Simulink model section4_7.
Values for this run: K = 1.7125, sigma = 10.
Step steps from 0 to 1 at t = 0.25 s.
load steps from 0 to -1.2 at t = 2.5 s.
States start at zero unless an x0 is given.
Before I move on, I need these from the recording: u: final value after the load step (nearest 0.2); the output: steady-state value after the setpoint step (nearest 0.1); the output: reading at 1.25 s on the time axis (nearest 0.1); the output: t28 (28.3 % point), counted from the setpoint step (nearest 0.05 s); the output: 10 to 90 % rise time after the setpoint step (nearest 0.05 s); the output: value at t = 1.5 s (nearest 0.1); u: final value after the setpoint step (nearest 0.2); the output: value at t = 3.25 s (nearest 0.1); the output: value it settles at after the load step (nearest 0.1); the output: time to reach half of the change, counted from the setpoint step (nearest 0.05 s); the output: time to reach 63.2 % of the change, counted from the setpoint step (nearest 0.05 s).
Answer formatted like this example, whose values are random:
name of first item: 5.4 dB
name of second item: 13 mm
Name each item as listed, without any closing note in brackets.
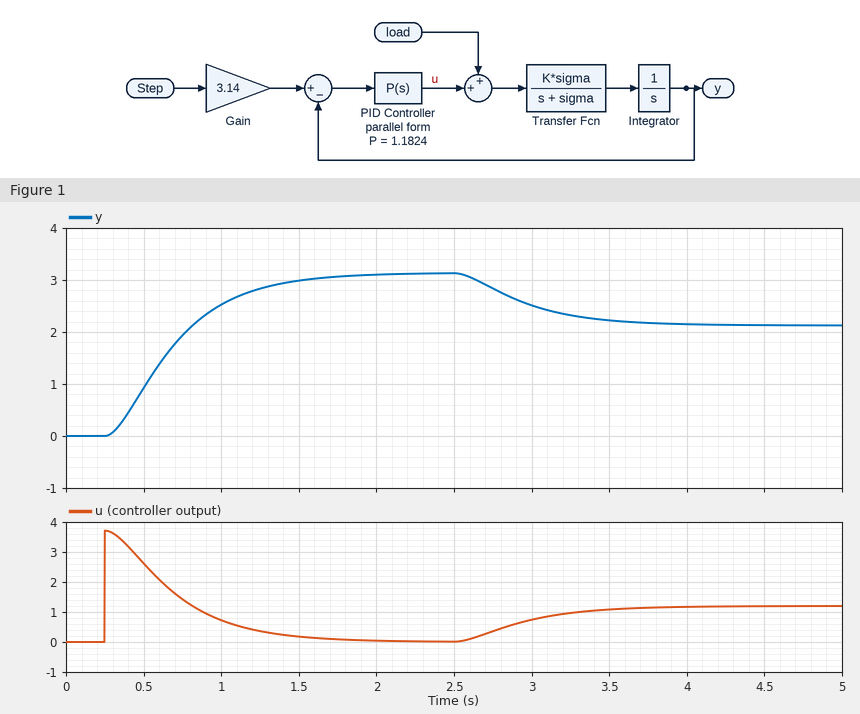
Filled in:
u: final value after the load step: 1.2
the output: steady-state value after the setpoint step: 3.1
the output: reading at 1.25 s on the time axis: 2.8
the output: t28 (28.3 % point), counted from the setpoint step: 0.25 s
the output: 10 to 90 % rise time after the setpoint step: 0.85 s
the output: value at t = 1.5 s: 3.0
u: final value after the setpoint step: 0.0
the output: value at t = 3.25 s: 2.3
the output: value it settles at after the load step: 2.1
the output: time to reach half of the change, counted from the setpoint step: 0.40 s
the output: time to reach 63.2 % of the change, counted from the setpoint step: 0.50 s
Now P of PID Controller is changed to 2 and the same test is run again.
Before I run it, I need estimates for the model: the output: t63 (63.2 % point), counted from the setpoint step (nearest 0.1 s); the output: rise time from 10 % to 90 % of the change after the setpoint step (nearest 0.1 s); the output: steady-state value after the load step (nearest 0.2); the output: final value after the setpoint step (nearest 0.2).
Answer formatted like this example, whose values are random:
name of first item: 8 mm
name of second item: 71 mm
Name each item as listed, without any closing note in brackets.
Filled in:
the output: t63 (63.2 % point), counted from the setpoint step: 0.3 s
the output: rise time from 10 % to 90 % of the change after the setpoint step: 0.5 s
the output: steady-state value after the load step: 2.6
the output: final value after the setpoint step: 3.2
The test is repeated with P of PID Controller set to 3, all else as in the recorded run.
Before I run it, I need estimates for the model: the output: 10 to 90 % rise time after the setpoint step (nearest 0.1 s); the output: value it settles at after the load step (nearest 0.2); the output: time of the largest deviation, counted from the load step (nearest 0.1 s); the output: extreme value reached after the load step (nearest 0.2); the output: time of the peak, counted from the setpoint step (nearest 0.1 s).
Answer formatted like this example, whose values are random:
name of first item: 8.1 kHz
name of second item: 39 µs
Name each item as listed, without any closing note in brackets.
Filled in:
the output: 10 to 90 % rise time after the setpoint step: 0.3 s
the output: value it settles at after the load step: 2.8
the output: time of the largest deviation, counted from the load step: 0.6 s
the output: extreme value reached after the load step: 2.8
the output: time of the peak, counted from the setpoint step: 0.6 s
